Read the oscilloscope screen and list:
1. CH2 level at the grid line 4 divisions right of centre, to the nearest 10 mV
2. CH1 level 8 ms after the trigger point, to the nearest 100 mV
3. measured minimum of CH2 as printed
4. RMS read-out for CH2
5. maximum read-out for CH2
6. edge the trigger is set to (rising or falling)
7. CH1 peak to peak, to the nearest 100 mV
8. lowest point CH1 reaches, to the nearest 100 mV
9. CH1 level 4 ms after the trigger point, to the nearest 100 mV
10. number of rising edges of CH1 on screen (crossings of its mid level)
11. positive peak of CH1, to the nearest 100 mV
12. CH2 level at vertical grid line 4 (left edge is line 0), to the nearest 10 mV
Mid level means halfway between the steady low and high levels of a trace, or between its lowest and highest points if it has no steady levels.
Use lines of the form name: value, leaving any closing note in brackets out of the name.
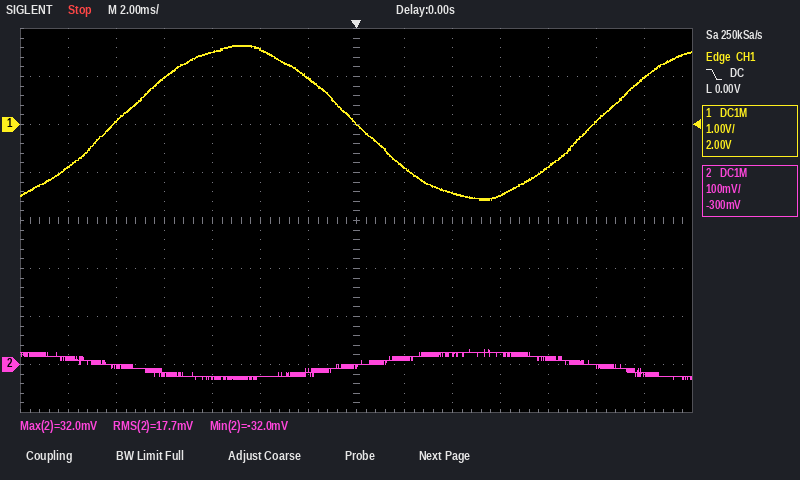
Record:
CH2 level at the grid line 4 divisions right of centre, to the nearest 10 mV: 10 mV
CH1 level 8 ms after the trigger point, to the nearest 100 mV: -900 mV
measured minimum of CH2 as printed: -32.0 mV
RMS read-out for CH2: 17.7 mV
maximum read-out for CH2: 32.0 mV
edge the trigger is set to: falling
CH1 peak to peak, to the nearest 100 mV: 3.2 V
lowest point CH1 reaches, to the nearest 100 mV: -1.6 V
CH1 level 4 ms after the trigger point, to the nearest 100 mV: -1.4 V
number of rising edges of CH1 on screen: 2
positive peak of CH1, to the nearest 100 mV: 1.6 V
CH2 level at vertical grid line 4 (left edge is line 0), to the nearest 10 mV: -30 mV
